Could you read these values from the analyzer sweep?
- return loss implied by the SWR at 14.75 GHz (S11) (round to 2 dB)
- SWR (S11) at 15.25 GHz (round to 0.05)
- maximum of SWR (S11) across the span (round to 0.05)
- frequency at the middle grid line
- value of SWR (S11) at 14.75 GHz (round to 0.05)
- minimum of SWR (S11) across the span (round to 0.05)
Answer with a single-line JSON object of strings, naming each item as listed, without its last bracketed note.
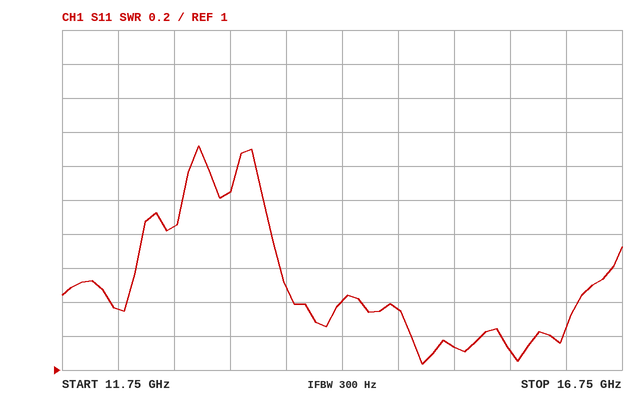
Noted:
{"return loss implied by the SWR at 14.75 GHz (S11)": "16 dB", "SWR (S11) at 15.25 GHz": "1.15", "maximum of SWR (S11) across the span": "2.30", "frequency at the middle grid line": "14.25 GHz", "value of SWR (S11) at 14.75 GHz": "1.35", "minimum of SWR (S11) across the span": "1.05"}
